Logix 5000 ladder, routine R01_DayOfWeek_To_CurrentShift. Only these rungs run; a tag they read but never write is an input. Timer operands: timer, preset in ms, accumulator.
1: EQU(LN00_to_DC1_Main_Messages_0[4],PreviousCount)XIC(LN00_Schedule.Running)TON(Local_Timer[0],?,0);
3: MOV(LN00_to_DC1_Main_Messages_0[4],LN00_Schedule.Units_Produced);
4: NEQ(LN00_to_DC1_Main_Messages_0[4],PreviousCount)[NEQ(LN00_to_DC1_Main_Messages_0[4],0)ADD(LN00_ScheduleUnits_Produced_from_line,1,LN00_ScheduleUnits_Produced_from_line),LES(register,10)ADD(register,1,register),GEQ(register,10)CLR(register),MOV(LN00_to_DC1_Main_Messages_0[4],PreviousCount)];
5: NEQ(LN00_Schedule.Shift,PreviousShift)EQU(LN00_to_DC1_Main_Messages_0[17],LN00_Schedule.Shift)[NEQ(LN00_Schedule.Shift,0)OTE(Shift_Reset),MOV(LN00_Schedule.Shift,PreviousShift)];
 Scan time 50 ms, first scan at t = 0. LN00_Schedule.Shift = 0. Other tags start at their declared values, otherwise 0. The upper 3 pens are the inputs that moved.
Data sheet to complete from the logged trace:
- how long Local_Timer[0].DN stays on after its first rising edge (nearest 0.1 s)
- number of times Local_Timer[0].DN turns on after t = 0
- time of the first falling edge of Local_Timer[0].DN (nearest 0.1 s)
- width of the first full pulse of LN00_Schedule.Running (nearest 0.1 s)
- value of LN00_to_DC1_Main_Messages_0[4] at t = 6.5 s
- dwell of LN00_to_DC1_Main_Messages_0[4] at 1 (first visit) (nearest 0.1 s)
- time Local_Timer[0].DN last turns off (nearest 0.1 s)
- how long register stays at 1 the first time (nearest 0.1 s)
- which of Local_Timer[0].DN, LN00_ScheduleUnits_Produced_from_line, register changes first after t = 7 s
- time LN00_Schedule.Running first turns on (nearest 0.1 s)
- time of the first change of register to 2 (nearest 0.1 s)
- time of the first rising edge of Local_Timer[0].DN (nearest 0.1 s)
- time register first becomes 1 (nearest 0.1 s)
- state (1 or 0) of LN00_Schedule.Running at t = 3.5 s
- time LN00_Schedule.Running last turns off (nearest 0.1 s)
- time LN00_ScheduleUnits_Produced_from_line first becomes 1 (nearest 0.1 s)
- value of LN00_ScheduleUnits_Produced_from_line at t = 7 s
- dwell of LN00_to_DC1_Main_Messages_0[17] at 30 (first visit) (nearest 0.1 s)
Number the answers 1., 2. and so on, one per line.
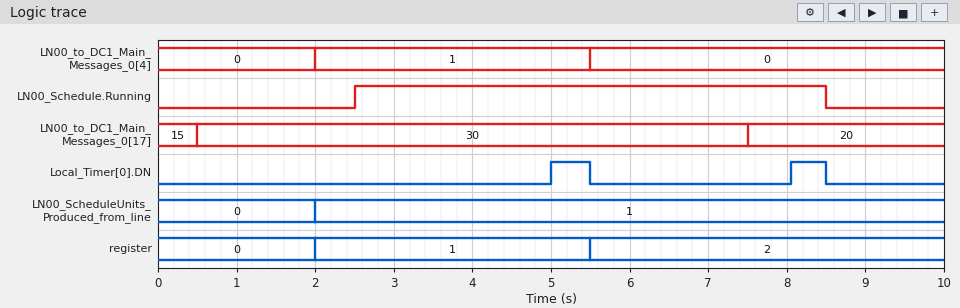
1. 0.5 s
2. 2
3. 5.5 s
4. 6.0 s
5. 0
6. 3.5 s
7. 8.5 s
8. 3.5 s
9. Local_Timer[0].DN
10. 2.5 s
11. 5.5 s
12. 5.0 s
13. 2.0 s
14. 1
15. 8.5 s
16. 2.0 s
17. 1
18. 7.0 s
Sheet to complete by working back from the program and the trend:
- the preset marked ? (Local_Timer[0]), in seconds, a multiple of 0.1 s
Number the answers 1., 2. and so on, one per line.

1. 2.5 s
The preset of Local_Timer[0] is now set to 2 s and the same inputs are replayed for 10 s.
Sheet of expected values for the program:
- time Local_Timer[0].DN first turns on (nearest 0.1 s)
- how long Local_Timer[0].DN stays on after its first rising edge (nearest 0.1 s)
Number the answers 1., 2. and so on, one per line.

1. 4.5 s
2. 1.0 s
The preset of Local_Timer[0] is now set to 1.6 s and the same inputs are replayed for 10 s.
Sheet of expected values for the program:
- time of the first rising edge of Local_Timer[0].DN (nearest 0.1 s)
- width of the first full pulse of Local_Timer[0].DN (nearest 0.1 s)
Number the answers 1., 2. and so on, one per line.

1. 4.1 s
2. 1.4 s
